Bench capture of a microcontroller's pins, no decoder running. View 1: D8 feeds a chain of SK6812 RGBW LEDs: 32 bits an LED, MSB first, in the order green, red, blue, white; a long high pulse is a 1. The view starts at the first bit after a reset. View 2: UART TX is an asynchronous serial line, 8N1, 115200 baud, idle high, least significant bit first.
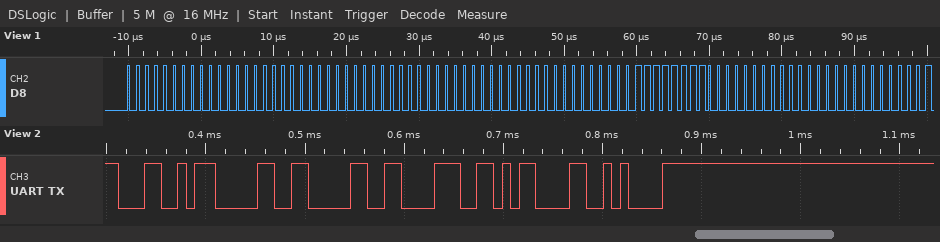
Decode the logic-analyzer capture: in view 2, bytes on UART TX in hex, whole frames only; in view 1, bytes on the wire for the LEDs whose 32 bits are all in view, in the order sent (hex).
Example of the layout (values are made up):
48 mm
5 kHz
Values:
0x4C 0x30 0x30 0x38 0x0D 0x0A
00 00 00 00 00 00 00 FF
